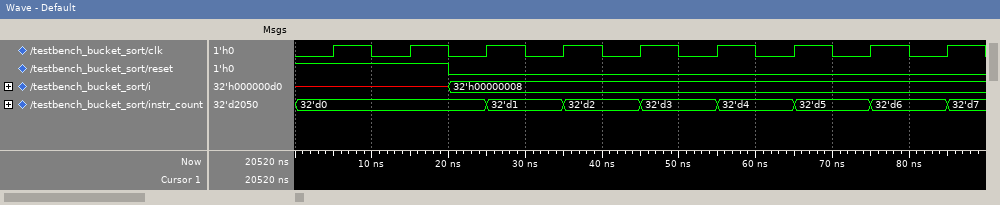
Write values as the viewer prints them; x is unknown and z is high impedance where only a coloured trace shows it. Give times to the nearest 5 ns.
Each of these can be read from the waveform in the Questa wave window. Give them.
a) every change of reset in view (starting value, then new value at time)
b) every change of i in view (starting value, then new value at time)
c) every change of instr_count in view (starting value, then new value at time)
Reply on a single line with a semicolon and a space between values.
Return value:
1, 0 at 20 ns; x, 32'h00000008 at 20 ns; 32'd0, 32'd1 at 25 ns, 32'd2 at 35 ns, 32'd3 at 45 ns, 32'd4 at 55 ns, 32'd5 at 65 ns, 32'd6 at 75 ns, 32'd7 at 85 ns
